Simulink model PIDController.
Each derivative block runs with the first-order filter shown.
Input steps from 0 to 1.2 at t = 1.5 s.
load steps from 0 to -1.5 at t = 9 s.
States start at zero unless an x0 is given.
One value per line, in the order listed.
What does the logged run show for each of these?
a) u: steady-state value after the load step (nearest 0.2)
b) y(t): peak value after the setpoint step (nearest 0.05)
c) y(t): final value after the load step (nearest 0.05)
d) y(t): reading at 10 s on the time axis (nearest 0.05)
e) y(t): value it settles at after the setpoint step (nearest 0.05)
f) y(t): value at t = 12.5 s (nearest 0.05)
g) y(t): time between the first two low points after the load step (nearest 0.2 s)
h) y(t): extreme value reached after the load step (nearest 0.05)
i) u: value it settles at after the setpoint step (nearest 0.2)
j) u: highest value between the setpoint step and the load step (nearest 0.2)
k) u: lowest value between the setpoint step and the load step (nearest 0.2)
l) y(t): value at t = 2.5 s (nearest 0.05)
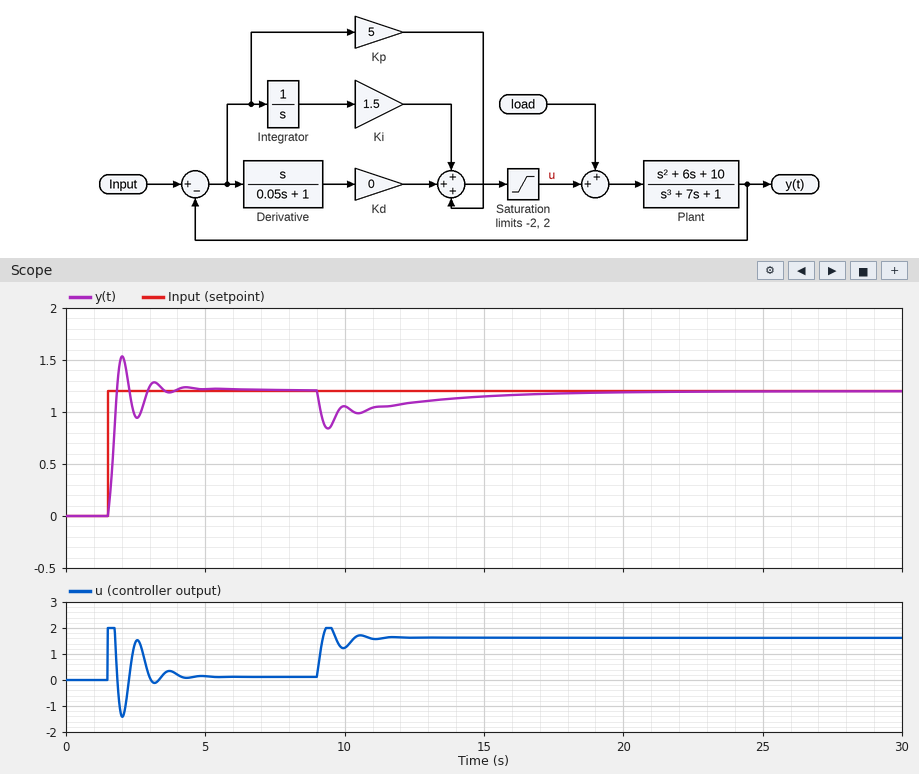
1.6
1.55
1.20
1.05
1.20
1.10
1.0 s
0.85
0.2
2.0
-1.4
0.95
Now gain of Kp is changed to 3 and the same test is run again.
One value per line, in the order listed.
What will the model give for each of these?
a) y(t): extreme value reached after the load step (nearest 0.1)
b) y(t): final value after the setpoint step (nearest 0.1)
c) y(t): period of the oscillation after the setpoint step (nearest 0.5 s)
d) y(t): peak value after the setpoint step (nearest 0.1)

0.6
1.2
1.5 s
1.6
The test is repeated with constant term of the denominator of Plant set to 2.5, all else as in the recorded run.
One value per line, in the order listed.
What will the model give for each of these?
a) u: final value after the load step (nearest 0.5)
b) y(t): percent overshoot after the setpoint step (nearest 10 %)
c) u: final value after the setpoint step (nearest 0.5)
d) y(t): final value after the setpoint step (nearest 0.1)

2.0
30 %
0.5
1.2
